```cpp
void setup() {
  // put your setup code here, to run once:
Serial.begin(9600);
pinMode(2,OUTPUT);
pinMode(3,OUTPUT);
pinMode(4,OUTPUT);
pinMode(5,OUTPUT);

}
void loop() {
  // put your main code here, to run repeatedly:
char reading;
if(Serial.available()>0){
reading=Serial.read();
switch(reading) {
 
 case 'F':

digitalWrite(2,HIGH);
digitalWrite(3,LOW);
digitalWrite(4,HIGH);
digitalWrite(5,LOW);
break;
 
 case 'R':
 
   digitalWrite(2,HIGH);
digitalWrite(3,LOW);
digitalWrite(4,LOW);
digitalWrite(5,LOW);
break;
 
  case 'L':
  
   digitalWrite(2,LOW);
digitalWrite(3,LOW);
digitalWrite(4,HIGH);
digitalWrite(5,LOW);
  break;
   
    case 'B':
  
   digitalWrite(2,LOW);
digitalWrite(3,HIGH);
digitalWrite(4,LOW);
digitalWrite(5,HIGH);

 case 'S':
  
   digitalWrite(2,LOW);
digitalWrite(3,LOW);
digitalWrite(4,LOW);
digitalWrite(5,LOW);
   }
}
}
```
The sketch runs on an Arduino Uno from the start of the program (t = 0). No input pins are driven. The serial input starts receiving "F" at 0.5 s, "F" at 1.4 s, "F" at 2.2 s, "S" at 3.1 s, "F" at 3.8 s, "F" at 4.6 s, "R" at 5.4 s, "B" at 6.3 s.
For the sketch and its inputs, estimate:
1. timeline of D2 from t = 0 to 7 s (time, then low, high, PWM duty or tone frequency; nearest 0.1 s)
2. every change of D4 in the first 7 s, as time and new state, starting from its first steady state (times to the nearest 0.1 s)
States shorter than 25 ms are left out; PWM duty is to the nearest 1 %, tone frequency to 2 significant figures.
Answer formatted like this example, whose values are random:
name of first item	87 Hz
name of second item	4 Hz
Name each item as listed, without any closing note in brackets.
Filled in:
timeline of D2 from t = 0 to 7 s	0 s low; 0.5 s high; 3.1 s low; 3.8 s high; 6.3 s low
every change of D4 in the first 7 s, as time and new state, starting from its first steady state	0 s low; 0.5 s high; 3.1 s low; 3.8 s high; 5.4 s low
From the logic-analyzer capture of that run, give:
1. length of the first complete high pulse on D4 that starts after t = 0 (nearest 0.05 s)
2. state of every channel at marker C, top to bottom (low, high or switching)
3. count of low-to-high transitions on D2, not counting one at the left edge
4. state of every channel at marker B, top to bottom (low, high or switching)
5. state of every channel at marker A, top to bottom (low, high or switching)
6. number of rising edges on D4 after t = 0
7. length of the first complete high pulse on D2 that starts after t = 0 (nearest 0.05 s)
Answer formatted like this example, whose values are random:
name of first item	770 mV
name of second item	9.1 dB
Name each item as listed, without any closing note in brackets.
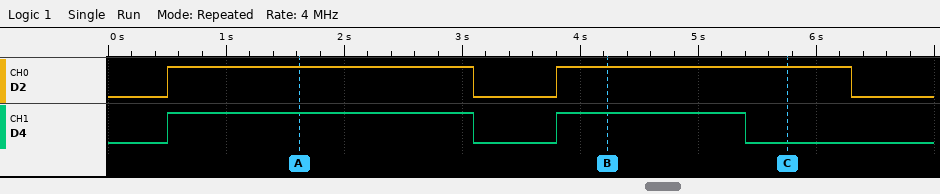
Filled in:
length of the first complete high pulse on D4 that starts after t = 0	2.60 s
state of every channel at marker C, top to bottom	D2 high, D4 low
count of low-to-high transitions on D2, not counting one at the left edge	2
state of every channel at marker B, top to bottom	D2 high, D4 high
state of every channel at marker A, top to bottom	D2 high, D4 high
number of rising edges on D4 after t = 0	2
length of the first complete high pulse on D2 that starts after t = 0	2.60 s
